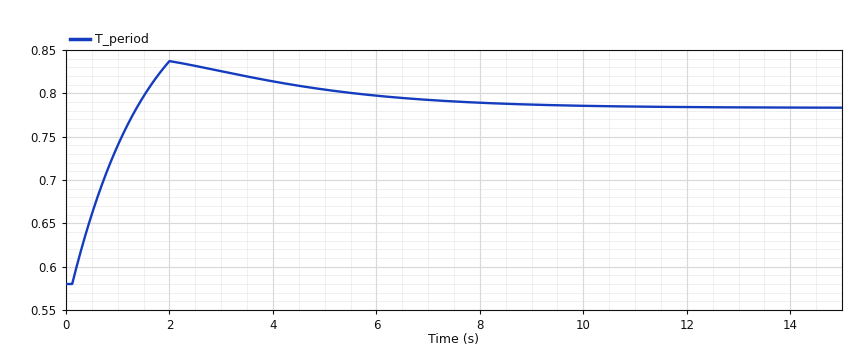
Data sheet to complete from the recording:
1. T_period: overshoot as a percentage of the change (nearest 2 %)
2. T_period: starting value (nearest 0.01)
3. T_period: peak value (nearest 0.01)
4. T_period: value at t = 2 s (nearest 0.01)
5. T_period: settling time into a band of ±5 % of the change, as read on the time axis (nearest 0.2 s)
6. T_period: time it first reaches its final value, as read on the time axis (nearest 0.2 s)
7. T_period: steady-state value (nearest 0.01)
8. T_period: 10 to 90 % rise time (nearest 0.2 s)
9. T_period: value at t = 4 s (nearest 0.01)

26 %
0.58
0.84
0.84
6.8 s
1.4 s
0.78
1.0 s
0.81
